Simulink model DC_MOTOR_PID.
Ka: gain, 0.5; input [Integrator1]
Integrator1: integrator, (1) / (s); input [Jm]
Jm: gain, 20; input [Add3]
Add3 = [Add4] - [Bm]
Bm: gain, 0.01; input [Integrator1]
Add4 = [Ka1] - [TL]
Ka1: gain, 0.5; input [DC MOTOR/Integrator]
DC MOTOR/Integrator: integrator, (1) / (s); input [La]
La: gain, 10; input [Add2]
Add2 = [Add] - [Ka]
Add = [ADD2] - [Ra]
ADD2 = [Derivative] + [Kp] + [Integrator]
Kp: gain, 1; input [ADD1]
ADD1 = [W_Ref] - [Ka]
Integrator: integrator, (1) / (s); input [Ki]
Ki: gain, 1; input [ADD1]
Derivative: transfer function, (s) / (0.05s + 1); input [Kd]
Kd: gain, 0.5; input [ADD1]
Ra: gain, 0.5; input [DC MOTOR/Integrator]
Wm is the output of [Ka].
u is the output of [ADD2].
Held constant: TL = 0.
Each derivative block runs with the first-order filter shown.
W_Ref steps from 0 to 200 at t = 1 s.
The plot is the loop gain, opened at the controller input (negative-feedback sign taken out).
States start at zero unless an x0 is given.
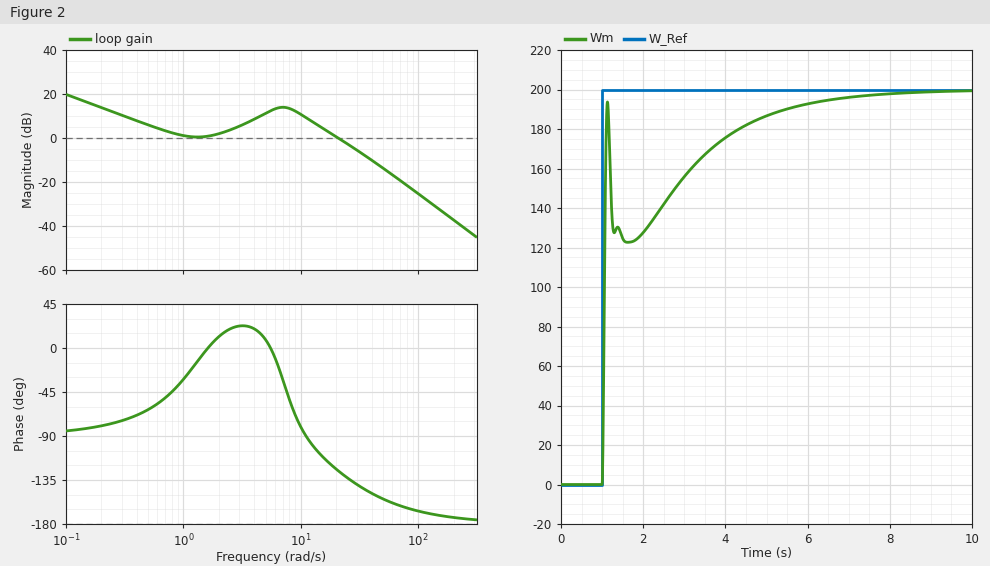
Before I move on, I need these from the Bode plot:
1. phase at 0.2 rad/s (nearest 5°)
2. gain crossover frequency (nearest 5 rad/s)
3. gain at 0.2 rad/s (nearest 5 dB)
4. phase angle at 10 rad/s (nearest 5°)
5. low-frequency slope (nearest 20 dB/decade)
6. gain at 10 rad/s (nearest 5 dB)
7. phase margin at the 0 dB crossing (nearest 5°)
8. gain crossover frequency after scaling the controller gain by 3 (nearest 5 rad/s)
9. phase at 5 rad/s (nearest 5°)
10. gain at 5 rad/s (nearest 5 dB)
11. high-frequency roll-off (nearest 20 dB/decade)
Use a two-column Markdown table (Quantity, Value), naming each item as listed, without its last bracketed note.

| Quantity | Value |
|---|---|
| phase at 0.2 rad/s | -80° |
| gain crossover frequency | 20 rad/s |
| gain at 0.2 rad/s | 15 dB |
| phase angle at 10 rad/s | -80° |
| low-frequency slope | -20 dB/decade |
| gain at 10 rad/s | 10 dB |
| phase margin at the 0 dB crossing | 55° |
| gain crossover frequency after scaling the controller gain by 3 | 40 rad/s |
| phase at 5 rad/s | 10° |
| gain at 5 rad/s | 10 dB |
| high-frequency roll-off | -40 dB/decade |
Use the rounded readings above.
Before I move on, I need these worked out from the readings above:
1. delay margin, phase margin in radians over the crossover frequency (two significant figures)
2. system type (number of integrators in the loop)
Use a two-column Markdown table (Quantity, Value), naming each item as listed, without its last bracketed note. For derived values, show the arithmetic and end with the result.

| Quantity | Value |
|---|---|
| delay margin, phase margin in radians over the crossover frequency | 55 × π / 180 / 20 = 0.048 s |
| system type | 1 |
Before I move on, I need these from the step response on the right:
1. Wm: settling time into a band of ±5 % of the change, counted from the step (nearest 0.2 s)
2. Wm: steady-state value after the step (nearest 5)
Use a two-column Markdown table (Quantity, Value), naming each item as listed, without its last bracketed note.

| Quantity | Value |
|---|---|
| Wm: settling time into a band of ±5 % of the change, counted from the step | 4.4 s |
| Wm: steady-state value after the step | 200 |
